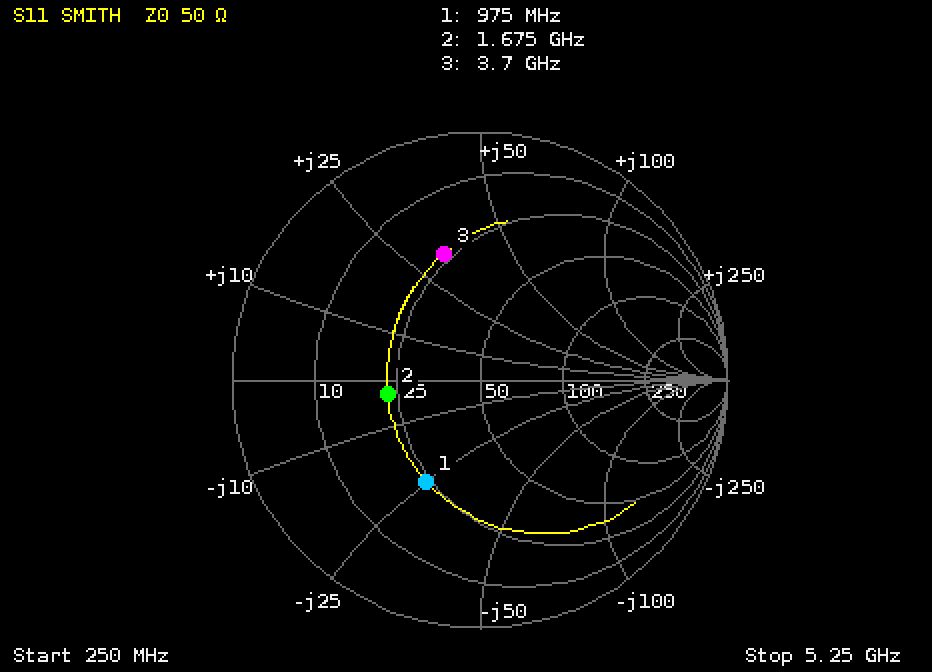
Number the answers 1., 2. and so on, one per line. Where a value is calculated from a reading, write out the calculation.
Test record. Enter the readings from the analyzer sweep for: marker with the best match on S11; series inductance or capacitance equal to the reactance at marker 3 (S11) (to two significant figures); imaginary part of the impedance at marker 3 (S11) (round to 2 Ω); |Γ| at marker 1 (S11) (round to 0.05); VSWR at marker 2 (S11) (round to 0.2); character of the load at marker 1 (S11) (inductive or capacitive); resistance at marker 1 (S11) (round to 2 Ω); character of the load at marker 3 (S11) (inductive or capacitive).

1. marker 2
2. L = 32 Ω/(2π × 3.7 GHz) ≈ 1.4 nH
3. +32 Ω
4. 0.45
5. 2.2
6. capacitive
7. 24 Ω
8. inductive
